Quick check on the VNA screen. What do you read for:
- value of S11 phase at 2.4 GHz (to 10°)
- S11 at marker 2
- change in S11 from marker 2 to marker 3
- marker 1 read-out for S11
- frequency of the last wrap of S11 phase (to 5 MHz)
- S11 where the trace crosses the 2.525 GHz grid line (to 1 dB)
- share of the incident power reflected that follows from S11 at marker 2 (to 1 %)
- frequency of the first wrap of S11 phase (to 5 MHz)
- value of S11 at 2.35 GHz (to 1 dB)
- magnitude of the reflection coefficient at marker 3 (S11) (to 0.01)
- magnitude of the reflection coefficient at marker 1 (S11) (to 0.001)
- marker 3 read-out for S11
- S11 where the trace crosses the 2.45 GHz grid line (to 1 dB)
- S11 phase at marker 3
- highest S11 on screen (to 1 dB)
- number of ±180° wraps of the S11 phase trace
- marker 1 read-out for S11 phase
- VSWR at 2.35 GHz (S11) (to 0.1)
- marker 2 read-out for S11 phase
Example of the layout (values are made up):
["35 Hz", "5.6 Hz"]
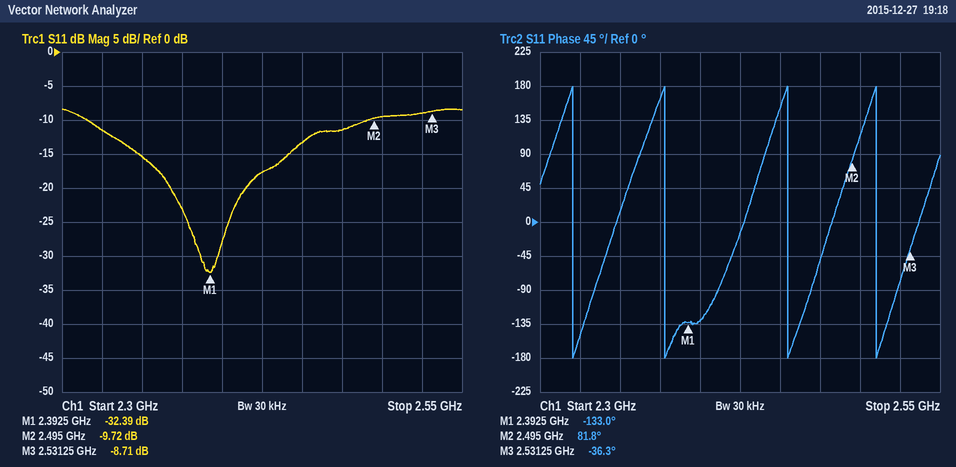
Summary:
["-130°", "-9.72 dB", "1.01 dB", "-32.39 dB", "2.510 GHz", "-9 dB", "11 %", "2.320 GHz", "-15 dB", "0.37", "0.024", "-8.71 dB", "-13 dB", "-36.3°", "-8 dB", "4", "-133.0°", "1.4", "81.8°"]
